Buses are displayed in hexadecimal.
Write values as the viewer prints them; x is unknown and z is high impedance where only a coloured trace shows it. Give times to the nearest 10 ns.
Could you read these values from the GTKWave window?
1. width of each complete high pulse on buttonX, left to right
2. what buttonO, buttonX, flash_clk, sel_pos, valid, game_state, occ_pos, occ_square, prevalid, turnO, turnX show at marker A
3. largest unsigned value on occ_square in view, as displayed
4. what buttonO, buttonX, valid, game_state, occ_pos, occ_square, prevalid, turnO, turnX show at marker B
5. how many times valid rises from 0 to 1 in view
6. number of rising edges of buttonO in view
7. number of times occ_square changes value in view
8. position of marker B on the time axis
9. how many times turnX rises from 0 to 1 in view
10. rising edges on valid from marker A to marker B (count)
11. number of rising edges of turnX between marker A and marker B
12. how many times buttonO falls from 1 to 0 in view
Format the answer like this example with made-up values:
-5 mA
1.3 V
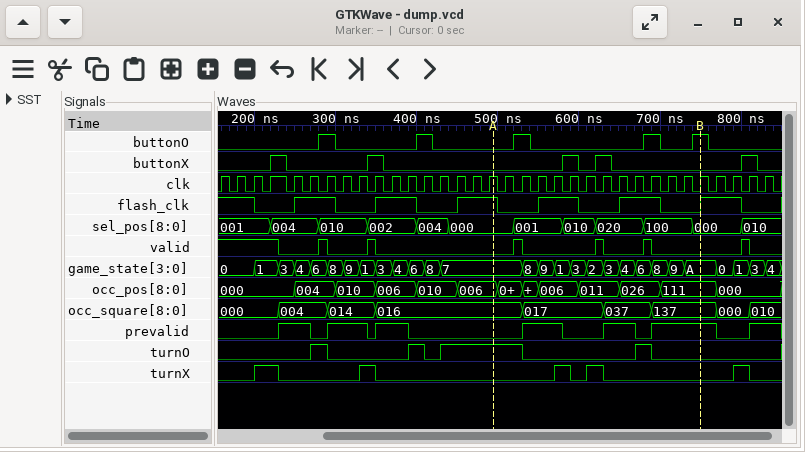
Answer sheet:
20 ns, 20 ns, 20 ns, 20 ns, 20 ns
buttonO=0, buttonX=0, flash_clk=1, sel_pos=000, valid=0, game_state=7, occ_pos=006, occ_square=016, prevalid=0, turnO=1, turnX=0
137
buttonO=1, buttonX=0, valid=0, game_state=A, occ_pos=111, occ_square=137, prevalid=1, turnO=0, turnX=0
6
5
8
750 ns
5
3
2
5
